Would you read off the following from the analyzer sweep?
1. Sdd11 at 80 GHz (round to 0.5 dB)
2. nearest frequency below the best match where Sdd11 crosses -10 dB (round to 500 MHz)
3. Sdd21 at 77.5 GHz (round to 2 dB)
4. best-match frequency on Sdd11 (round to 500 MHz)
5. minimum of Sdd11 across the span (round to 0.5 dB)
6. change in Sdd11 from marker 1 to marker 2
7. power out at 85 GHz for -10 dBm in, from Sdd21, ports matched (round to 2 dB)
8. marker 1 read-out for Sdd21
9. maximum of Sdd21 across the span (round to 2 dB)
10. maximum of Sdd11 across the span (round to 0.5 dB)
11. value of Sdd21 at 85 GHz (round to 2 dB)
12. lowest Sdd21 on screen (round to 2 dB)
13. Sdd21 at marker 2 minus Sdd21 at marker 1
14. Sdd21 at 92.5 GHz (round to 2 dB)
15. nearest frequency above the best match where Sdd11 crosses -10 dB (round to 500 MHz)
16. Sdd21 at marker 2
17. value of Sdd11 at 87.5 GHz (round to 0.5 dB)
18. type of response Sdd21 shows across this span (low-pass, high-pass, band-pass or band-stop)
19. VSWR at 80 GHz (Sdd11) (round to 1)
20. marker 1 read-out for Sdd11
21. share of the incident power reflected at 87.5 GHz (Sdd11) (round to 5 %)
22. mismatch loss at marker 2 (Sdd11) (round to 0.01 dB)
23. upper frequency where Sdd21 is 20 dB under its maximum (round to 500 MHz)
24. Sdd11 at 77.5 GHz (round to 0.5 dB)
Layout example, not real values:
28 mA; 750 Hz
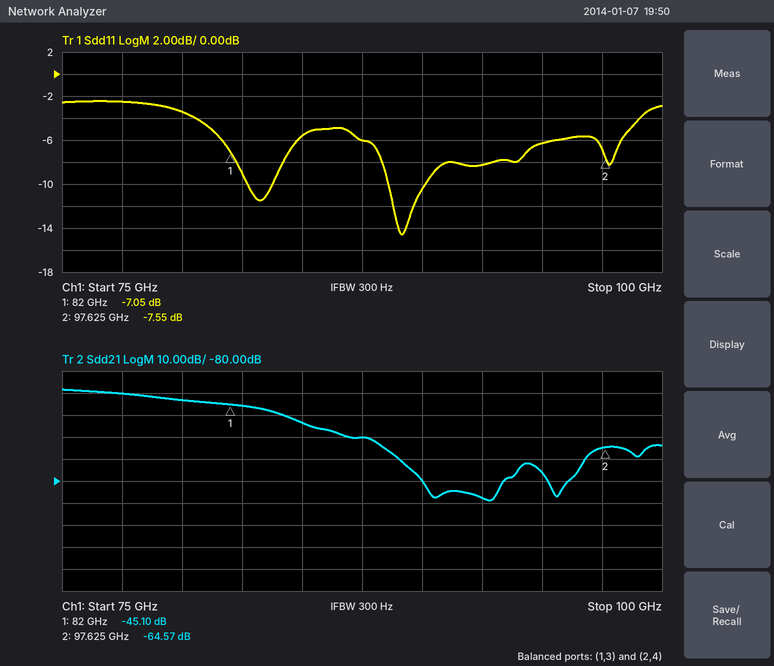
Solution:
-3.5 dB; 88.5 GHz; -40 dB; 89.0 GHz; -14.5 dB; -0.50 dB; -64 dBm; -45.10 dB; -38 dB; -2.5 dB; -54 dB; -88 dB; -19.47 dB; -88 dB; 90.0 GHz; -64.57 dB; -6.0 dB; low-pass; 5; -7.05 dB; 25 %; 0.84 dB; 86.5 GHz; -2.5 dB
